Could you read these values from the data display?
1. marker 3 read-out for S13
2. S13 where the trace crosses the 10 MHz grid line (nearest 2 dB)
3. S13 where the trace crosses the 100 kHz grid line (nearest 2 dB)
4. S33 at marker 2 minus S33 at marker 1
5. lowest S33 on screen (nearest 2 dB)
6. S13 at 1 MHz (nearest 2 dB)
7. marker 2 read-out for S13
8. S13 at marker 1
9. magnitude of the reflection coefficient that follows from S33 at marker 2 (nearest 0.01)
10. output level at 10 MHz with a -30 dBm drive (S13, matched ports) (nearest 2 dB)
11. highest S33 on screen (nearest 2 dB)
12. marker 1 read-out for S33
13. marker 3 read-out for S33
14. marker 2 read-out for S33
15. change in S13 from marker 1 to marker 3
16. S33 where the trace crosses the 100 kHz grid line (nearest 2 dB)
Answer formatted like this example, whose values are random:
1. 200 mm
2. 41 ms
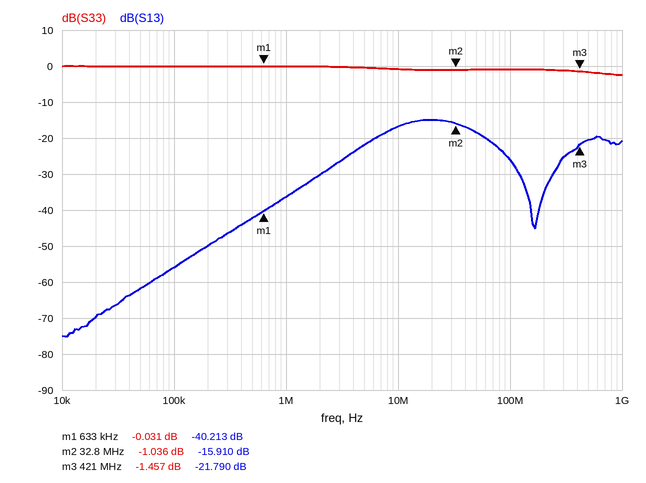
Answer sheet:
1. -21.790 dB
2. -16 dB
3. -56 dB
4. -1.005 dB
5. -2 dB
6. -36 dB
7. -15.910 dB
8. -40.213 dB
9. 0.89
10. -46 dBm
11. 0 dB
12. -0.031 dB
13. -1.457 dB
14. -1.036 dB
15. 18.423 dB
16. 0 dB
